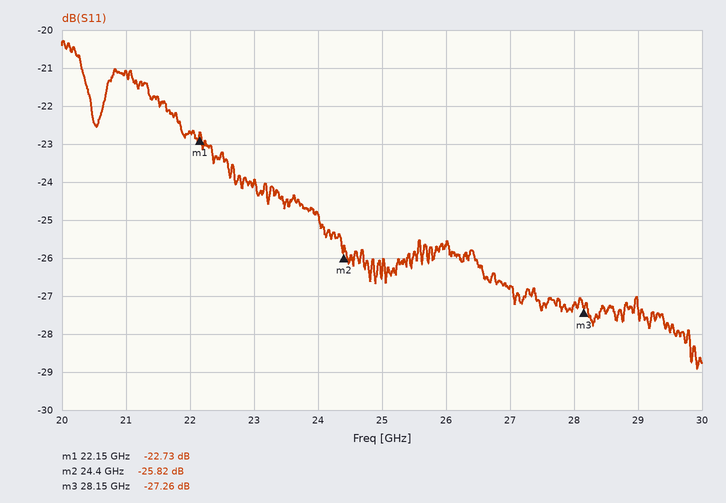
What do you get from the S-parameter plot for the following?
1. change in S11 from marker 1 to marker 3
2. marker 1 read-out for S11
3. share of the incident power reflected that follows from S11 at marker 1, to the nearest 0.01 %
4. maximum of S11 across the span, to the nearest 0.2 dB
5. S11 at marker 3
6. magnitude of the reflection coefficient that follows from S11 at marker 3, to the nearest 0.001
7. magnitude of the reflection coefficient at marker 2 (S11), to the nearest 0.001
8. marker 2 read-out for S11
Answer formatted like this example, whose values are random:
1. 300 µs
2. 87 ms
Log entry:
1. -4.53 dB
2. -22.73 dB
3. 0.53 %
4. -20.2 dB
5. -27.26 dB
6. 0.043
7. 0.051
8. -25.82 dB
